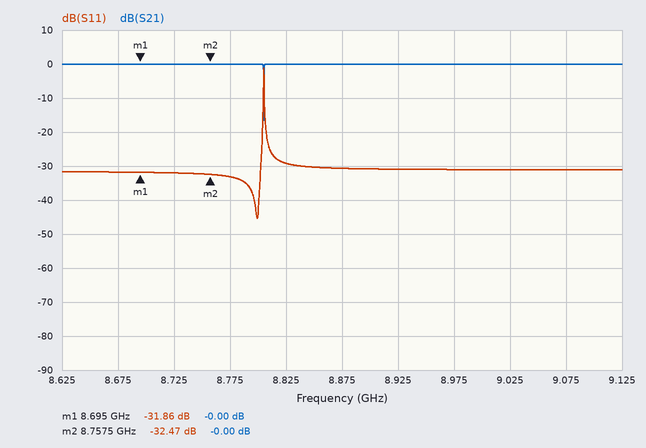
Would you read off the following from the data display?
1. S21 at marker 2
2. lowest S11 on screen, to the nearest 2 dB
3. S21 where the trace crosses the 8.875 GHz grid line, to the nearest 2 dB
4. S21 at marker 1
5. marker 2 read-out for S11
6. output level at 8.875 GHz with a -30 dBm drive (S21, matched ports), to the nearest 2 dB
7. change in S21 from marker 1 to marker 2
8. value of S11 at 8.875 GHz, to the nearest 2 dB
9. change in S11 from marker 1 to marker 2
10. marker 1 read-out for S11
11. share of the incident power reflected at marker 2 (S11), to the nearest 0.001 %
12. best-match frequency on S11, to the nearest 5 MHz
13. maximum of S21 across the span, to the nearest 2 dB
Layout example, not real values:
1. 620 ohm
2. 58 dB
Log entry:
1. -0.00 dB
2. -46 dB
3. 0 dB
4. -0.00 dB
5. -32.47 dB
6. -30 dBm
7. 0.00 dB
8. -30 dB
9. -0.61 dB
10. -31.86 dB
11. 0.057 %
12. 8.800 GHz
13. 0 dB
